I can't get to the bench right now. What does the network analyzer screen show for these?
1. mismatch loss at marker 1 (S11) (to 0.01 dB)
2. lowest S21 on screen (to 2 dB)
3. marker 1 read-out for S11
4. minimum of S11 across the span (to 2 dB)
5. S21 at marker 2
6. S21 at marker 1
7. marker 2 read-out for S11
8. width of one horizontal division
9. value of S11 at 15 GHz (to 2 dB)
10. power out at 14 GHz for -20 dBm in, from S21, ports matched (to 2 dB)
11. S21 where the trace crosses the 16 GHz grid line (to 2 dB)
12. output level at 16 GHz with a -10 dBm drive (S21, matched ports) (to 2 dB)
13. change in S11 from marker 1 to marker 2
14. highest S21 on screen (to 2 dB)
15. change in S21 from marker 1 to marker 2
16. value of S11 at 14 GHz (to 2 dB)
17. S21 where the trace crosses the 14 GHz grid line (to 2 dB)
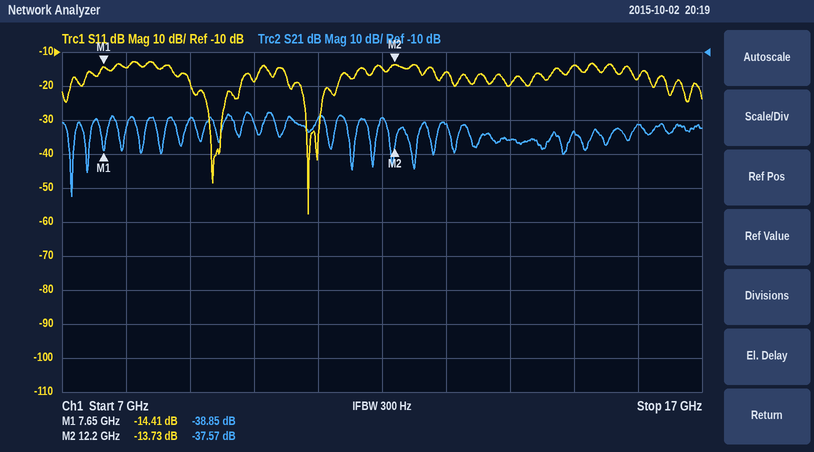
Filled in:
0.16 dB
-52 dB
-14.41 dB
-58 dB
-37.57 dB
-38.85 dB
-13.73 dB
1 GHz
-14 dB
-56 dBm
-32 dB
-42 dBm
0.68 dB
-28 dB
1.28 dB
-20 dB
-36 dB
